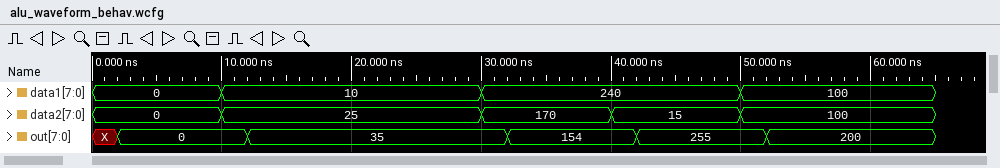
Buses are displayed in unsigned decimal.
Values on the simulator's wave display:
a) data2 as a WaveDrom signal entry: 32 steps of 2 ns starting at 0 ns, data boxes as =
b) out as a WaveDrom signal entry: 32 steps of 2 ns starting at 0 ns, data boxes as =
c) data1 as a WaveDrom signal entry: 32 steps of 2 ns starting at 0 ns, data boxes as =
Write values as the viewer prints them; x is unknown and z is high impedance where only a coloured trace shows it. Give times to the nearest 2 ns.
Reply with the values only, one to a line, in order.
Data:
{name: 'data2', wave: '=....=.........=....=....=......', data: '0 25 170 15 100'}
{name: 'out', wave: 'x=....=.........=....=....=.....', data: '0 35 154 255 200'}
{name: 'data1', wave: '=....=.........=.........=......', data: '0 10 240 100'}
